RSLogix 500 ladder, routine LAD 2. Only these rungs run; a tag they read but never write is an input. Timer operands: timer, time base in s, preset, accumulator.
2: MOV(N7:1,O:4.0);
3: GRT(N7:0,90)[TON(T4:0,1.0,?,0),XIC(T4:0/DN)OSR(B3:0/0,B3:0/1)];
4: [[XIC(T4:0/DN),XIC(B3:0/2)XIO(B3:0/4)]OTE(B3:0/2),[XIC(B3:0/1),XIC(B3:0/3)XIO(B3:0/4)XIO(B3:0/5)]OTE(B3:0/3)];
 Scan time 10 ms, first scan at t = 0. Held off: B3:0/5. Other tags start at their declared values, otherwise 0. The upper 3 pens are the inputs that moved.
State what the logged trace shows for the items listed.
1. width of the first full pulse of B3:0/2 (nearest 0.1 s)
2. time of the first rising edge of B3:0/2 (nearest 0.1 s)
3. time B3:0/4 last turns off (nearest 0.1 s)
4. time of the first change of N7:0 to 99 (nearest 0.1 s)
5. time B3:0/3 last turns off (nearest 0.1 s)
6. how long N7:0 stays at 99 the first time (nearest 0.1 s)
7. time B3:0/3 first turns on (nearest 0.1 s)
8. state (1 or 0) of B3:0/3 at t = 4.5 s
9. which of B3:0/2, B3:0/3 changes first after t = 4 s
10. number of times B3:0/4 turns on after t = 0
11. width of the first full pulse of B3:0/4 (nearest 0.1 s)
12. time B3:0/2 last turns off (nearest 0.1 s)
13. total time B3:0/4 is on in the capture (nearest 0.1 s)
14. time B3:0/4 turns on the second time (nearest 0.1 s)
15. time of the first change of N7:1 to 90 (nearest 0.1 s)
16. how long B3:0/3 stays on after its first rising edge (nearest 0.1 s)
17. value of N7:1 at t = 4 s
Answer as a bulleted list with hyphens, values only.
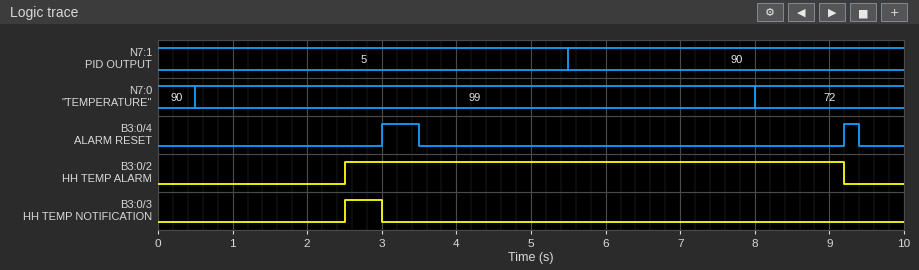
- 6.7 s
- 2.5 s
- 9.4 s
- 0.5 s
- 3.0 s
- 7.5 s
- 2.5 s
- 0
- B3:0/2
- 2
- 0.5 s
- 9.2 s
- 0.7 s
- 9.2 s
- 5.5 s
- 0.5 s
- 5
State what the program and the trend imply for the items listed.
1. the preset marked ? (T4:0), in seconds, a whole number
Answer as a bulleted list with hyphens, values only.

- 2 s
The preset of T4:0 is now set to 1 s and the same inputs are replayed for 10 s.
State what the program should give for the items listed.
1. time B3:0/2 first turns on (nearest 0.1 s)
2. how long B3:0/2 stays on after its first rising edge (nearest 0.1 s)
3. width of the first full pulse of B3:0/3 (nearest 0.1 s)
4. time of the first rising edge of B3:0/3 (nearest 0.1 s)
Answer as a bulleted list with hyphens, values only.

- 1.5 s
- 7.7 s
- 1.5 s
- 1.5 s
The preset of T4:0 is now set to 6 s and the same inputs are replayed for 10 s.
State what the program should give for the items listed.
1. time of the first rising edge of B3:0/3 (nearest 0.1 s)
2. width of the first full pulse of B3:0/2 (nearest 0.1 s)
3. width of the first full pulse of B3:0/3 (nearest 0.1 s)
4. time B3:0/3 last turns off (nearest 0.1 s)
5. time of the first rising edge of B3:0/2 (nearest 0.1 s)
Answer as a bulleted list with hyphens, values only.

- 6.5 s
- 2.7 s
- 2.7 s
- 9.2 s
- 6.5 s
